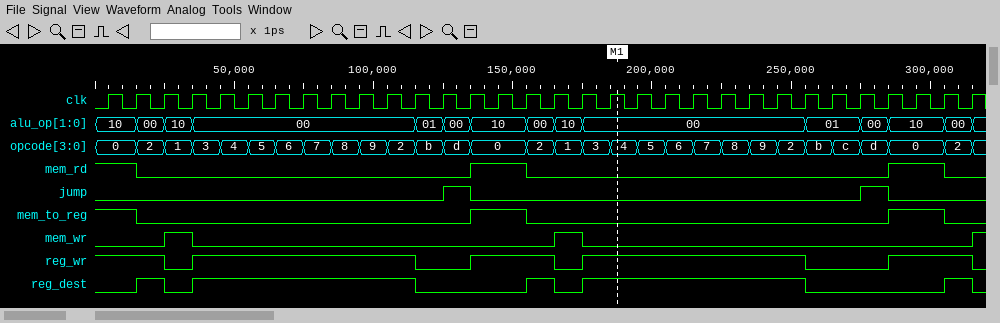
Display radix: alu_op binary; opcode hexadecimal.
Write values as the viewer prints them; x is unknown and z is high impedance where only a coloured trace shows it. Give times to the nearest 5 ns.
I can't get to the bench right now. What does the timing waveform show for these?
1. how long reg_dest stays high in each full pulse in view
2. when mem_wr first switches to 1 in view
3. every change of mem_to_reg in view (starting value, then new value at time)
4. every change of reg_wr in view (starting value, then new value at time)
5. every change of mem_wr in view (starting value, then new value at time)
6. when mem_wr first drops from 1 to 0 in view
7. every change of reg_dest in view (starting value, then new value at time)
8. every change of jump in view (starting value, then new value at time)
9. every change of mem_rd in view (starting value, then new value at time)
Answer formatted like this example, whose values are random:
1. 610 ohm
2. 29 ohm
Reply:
1. 10 ns, 80 ns, 10 ns, 80 ns, 10 ns
2. 25 ns
3. 1, 0 at 15 ns, 1 at 135 ns, 0 at 155 ns, 1 at 285 ns, 0 at 305 ns
4. 1, 0 at 25 ns, 1 at 35 ns, 0 at 115 ns, 1 at 135 ns, 0 at 165 ns, 1 at 175 ns, 0 at 255 ns, 1 at 285 ns, 0 at 315 ns
5. 0, 1 at 25 ns, 0 at 35 ns, 1 at 165 ns, 0 at 175 ns, 1 at 315 ns
6. 35 ns
7. 0, 1 at 15 ns, 0 at 25 ns, 1 at 35 ns, 0 at 115 ns, 1 at 155 ns, 0 at 165 ns, 1 at 175 ns, 0 at 255 ns, 1 at 305 ns, 0 at 315 ns
8. 0, 1 at 125 ns, 0 at 135 ns, 1 at 275 ns, 0 at 285 ns
9. 1, 0 at 15 ns, 1 at 135 ns, 0 at 155 ns, 1 at 285 ns, 0 at 305 ns
